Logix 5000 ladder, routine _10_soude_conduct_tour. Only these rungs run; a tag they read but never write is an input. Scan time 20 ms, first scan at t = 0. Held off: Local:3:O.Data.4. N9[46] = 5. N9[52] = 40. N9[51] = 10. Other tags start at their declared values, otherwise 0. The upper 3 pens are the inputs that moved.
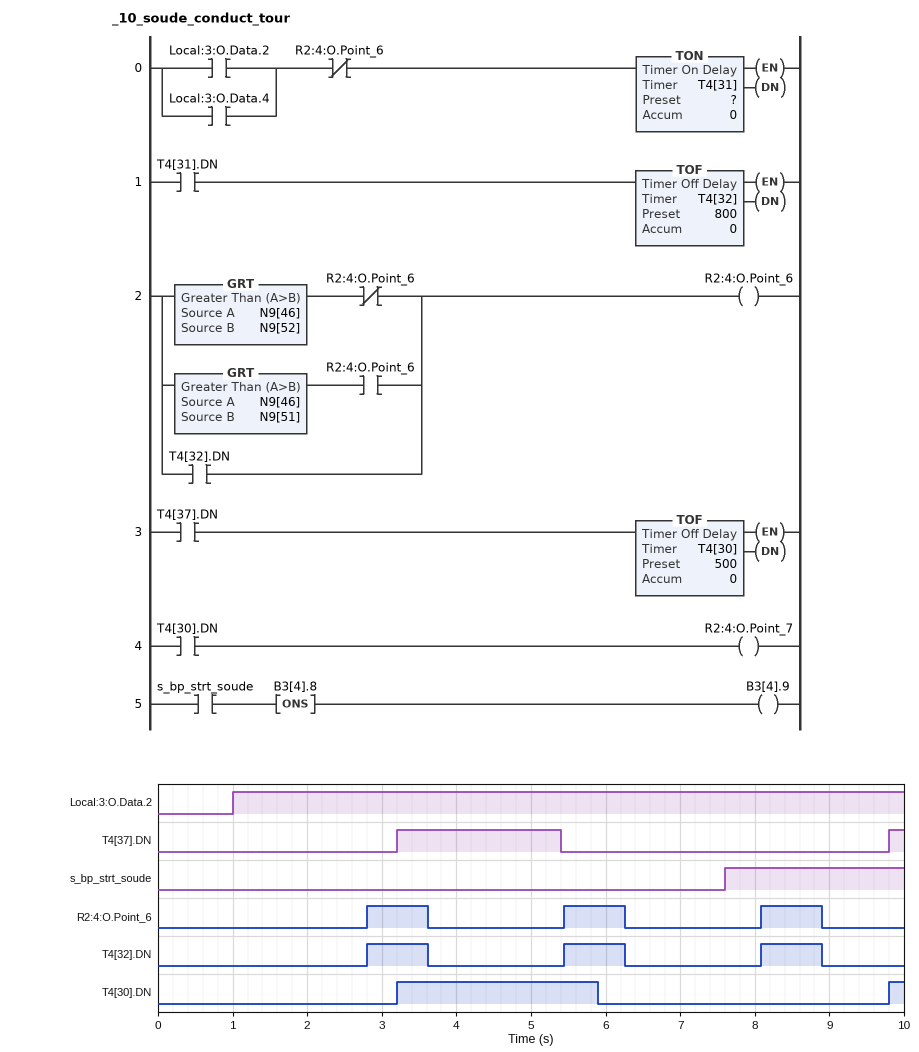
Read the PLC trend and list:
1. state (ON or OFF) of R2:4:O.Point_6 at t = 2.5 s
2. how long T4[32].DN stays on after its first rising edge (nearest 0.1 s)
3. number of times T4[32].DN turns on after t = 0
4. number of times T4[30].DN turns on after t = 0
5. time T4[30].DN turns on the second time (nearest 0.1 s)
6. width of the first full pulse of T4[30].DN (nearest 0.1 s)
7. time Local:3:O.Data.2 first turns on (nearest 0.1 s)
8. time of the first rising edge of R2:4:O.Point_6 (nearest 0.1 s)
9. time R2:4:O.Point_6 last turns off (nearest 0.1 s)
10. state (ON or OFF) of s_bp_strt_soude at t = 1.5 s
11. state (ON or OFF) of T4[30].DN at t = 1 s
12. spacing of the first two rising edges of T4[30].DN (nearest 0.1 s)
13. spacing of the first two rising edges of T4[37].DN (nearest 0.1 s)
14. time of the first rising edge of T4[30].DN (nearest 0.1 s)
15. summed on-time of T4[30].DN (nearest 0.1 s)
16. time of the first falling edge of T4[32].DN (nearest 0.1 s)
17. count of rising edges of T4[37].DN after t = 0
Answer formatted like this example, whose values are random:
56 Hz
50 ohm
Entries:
OFF
0.8 s
3
2
9.8 s
2.7 s
1.0 s
2.8 s
8.9 s
OFF
OFF
6.6 s
6.6 s
3.2 s
2.9 s
3.6 s
2
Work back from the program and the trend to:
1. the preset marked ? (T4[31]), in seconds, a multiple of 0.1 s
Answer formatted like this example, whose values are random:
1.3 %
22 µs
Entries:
1.8 s
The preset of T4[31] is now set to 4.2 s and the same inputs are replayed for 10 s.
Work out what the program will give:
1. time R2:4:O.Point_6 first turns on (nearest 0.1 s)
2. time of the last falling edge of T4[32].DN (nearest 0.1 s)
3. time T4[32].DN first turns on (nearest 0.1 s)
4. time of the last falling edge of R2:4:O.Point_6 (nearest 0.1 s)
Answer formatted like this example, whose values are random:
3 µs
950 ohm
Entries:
5.2 s
6.0 s
5.2 s
6.0 s
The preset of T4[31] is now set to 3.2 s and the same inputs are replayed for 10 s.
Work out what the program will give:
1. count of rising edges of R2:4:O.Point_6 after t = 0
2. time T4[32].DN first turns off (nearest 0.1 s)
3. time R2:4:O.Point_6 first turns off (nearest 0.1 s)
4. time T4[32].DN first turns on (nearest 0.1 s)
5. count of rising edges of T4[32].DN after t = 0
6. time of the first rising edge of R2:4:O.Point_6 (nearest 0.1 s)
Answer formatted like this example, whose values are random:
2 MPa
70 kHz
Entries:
2
5.0 s
5.0 s
4.2 s
2
4.2 s
